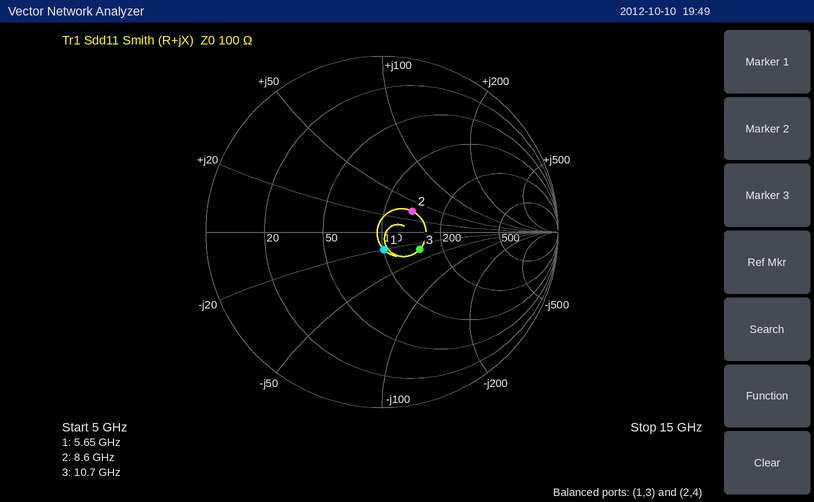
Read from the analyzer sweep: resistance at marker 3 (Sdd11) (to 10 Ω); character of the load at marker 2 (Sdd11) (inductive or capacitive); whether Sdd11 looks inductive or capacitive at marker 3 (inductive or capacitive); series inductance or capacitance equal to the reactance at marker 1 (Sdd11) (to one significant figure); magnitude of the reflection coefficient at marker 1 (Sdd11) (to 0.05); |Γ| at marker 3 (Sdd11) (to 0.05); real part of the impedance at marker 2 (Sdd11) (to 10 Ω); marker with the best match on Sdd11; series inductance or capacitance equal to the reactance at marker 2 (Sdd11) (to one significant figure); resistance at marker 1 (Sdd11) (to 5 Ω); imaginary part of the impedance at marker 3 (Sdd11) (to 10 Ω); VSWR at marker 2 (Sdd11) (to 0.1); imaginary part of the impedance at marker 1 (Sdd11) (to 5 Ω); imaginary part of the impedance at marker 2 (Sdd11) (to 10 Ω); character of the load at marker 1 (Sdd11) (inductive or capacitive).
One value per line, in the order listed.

150 Ω
inductive
capacitive
1 pF
0.10
0.25
140 Ω
marker 1
600 pH
100 Ω
-30 Ω
1.5
-20 Ω
+30 Ω
capacitive
